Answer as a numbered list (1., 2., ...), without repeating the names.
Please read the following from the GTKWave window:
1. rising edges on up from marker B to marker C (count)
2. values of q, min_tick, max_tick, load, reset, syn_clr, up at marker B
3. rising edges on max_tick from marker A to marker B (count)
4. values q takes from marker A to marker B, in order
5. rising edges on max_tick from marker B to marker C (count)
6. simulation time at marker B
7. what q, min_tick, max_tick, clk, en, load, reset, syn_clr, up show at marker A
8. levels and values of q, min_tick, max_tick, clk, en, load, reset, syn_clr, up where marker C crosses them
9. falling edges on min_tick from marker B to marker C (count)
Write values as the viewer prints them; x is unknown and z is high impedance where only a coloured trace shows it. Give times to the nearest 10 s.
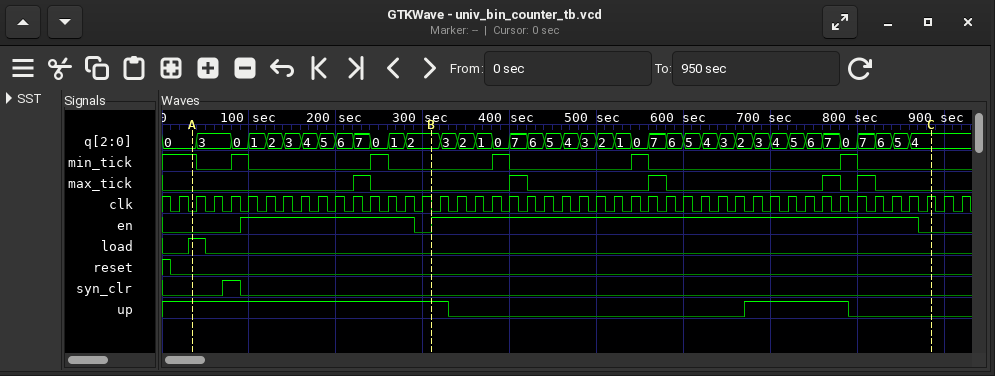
1. 1
2. q=2, min_tick=0, max_tick=0, load=0, reset=0, syn_clr=0, up=1
3. 1
4. 0, 3, 0, 1, 2, 3, 4, 5, 6, 7, 0, 1, 2
5. 4
6. 310 s
7. q=0, min_tick=1, max_tick=0, clk=0, en=0, load=1, reset=0, syn_clr=0, up=1
8. q=4, min_tick=0, max_tick=0, clk=1, en=0, load=0, reset=0, syn_clr=0, up=0
9. 3
